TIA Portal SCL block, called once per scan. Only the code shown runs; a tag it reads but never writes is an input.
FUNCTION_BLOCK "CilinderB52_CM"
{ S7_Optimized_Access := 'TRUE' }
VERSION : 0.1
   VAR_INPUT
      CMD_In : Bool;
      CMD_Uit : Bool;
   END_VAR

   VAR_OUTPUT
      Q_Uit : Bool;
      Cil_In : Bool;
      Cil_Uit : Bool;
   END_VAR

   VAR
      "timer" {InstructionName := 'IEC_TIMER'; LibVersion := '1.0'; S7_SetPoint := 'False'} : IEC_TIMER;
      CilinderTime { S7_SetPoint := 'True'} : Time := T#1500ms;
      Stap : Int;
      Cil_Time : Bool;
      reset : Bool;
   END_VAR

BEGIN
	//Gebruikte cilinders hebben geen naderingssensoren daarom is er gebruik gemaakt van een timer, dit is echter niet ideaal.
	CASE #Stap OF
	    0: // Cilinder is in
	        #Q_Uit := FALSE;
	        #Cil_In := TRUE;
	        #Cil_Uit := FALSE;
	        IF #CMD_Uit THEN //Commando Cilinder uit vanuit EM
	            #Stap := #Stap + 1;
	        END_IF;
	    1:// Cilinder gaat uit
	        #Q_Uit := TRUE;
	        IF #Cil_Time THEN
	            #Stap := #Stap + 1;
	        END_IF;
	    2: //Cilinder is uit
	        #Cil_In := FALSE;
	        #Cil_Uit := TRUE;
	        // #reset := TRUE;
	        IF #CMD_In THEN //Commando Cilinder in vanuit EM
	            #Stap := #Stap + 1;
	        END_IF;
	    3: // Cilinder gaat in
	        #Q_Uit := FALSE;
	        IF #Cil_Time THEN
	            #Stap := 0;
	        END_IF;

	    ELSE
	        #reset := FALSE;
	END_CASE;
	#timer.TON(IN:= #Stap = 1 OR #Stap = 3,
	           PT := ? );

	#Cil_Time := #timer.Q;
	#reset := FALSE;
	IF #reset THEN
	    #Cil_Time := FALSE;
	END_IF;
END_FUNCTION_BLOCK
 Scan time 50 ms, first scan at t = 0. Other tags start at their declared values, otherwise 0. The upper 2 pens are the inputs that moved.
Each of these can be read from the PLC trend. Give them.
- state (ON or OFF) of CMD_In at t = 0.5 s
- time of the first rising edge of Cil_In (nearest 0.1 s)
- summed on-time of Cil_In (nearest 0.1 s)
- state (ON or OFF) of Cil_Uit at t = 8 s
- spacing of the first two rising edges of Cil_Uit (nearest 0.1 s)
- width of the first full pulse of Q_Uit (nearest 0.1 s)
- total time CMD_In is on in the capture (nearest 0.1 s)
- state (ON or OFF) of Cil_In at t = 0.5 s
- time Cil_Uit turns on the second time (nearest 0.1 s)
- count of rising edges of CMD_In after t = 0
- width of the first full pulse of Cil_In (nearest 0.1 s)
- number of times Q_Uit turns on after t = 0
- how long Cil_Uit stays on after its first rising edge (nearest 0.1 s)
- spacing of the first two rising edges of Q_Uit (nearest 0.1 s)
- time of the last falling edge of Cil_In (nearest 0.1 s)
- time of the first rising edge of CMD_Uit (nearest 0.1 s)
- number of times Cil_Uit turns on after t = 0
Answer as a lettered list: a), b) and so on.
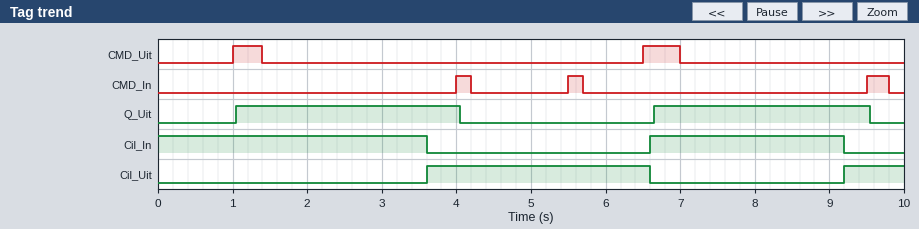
a) OFF
b) 6.6 s
c) 6.2 s
d) OFF
e) 5.6 s
f) 3.0 s
g) 0.7 s
h) ON
i) 9.2 s
j) 3
k) 2.6 s
l) 2
m) 3.0 s
n) 5.6 s
o) 9.2 s
p) 1.0 s
q) 2
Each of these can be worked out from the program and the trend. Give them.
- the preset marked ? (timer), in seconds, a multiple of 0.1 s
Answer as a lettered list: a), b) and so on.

a) 2.5 s
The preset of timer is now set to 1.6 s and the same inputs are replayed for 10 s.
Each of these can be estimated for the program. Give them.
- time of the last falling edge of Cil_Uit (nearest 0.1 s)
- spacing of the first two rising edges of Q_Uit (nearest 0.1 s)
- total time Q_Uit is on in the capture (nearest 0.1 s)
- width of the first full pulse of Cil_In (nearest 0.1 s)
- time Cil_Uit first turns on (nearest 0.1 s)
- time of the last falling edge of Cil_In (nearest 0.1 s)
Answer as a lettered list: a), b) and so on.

a) 5.7 s
b) 5.5 s
c) 6.0 s
d) 2.5 s
e) 2.7 s
f) 8.2 s
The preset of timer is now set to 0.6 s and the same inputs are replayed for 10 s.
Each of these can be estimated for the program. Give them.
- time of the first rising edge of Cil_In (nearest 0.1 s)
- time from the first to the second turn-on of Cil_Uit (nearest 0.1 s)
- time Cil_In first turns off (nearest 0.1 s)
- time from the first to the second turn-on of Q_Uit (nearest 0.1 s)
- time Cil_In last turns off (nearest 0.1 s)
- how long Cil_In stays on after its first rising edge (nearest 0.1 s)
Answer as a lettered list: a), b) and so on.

a) 4.7 s
b) 5.5 s
c) 1.7 s
d) 5.5 s
e) 7.2 s
f) 2.5 s
